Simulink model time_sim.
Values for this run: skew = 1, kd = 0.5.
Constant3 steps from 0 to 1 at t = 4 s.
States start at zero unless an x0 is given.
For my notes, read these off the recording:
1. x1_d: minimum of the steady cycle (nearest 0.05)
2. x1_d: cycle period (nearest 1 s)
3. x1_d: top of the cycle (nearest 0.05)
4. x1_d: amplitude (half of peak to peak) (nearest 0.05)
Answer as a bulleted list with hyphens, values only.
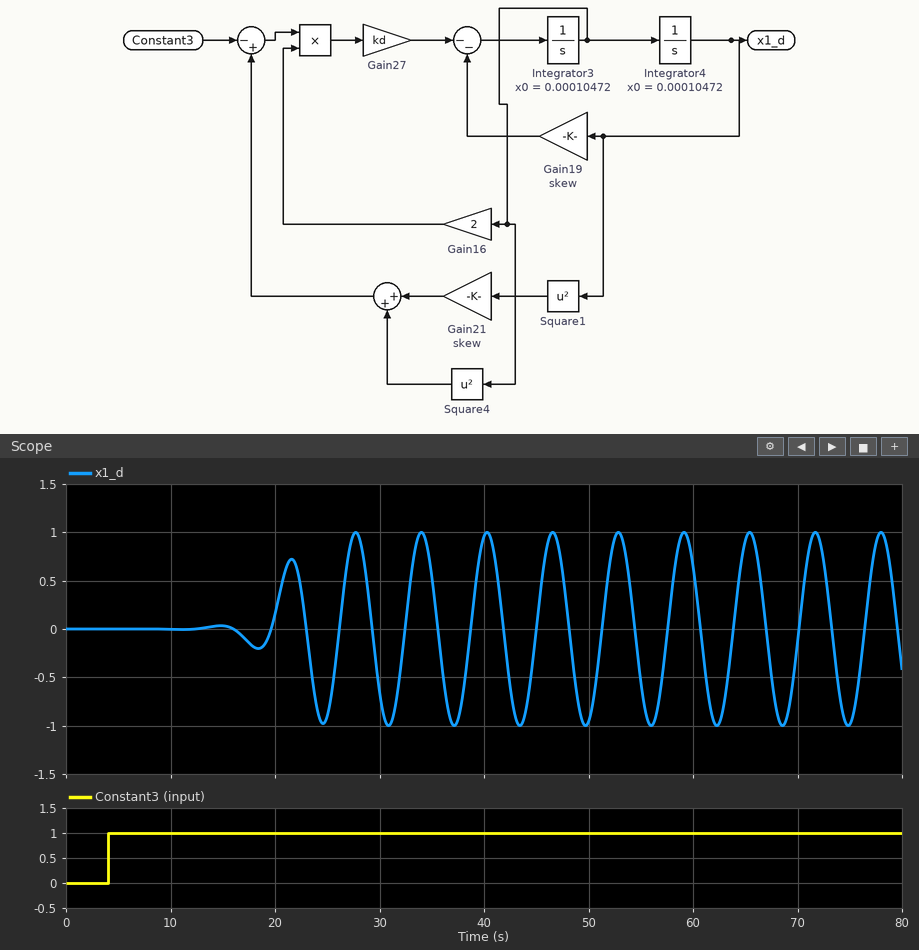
- -1.00
- 6 s
- 1.00
- 1.00
